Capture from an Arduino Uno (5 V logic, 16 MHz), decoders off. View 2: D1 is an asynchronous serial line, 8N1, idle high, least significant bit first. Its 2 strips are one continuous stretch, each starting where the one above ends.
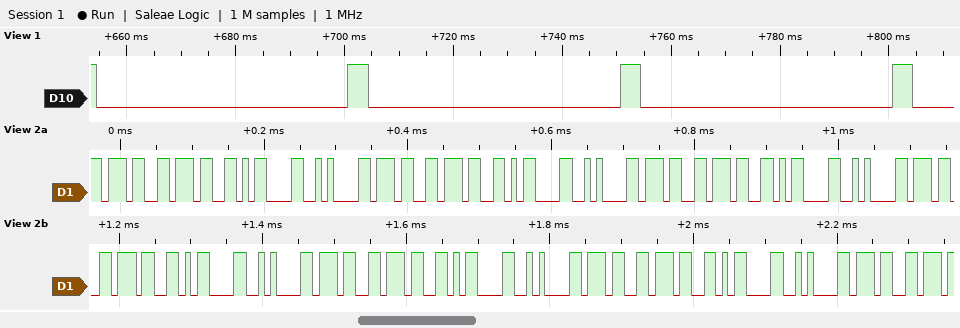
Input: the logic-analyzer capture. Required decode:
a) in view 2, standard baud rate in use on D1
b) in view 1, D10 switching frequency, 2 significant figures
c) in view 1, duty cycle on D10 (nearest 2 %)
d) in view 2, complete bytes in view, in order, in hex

115200 baud
20 Hz
8 %
37 37 0D 0A 37 37 0D 0A 37 37 0D 0A 37 37 0D 0A 37 37 0D 0A 37 37 0D 0A 37
